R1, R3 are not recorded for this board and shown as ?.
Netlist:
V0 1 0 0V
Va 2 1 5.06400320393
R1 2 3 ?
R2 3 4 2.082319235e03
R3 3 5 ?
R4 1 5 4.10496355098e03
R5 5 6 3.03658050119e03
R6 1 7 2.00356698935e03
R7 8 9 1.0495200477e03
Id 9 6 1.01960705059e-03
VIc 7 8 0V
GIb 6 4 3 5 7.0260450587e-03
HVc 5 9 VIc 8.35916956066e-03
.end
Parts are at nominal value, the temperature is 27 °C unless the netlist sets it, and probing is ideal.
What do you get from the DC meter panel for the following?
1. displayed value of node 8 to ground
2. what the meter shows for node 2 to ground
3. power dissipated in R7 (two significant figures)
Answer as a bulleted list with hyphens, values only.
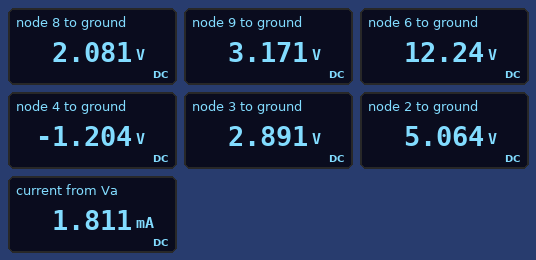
- 2.081 V
- 5.064 V
- 1.1 mW
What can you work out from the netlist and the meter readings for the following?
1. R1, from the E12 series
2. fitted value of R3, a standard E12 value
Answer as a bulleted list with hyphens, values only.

- 1.2 kΩ
- 1.8 kΩ
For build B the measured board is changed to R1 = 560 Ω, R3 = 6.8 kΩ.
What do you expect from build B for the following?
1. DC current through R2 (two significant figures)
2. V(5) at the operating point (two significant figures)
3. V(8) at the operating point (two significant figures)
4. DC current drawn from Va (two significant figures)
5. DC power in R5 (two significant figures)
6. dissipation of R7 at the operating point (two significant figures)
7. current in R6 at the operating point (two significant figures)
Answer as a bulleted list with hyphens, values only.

- 2.4 mA
- 4.1 V
- 2.7 V
- 2.3 mA
- 35 mW
- 1.9 mW
- 1.3 mA
